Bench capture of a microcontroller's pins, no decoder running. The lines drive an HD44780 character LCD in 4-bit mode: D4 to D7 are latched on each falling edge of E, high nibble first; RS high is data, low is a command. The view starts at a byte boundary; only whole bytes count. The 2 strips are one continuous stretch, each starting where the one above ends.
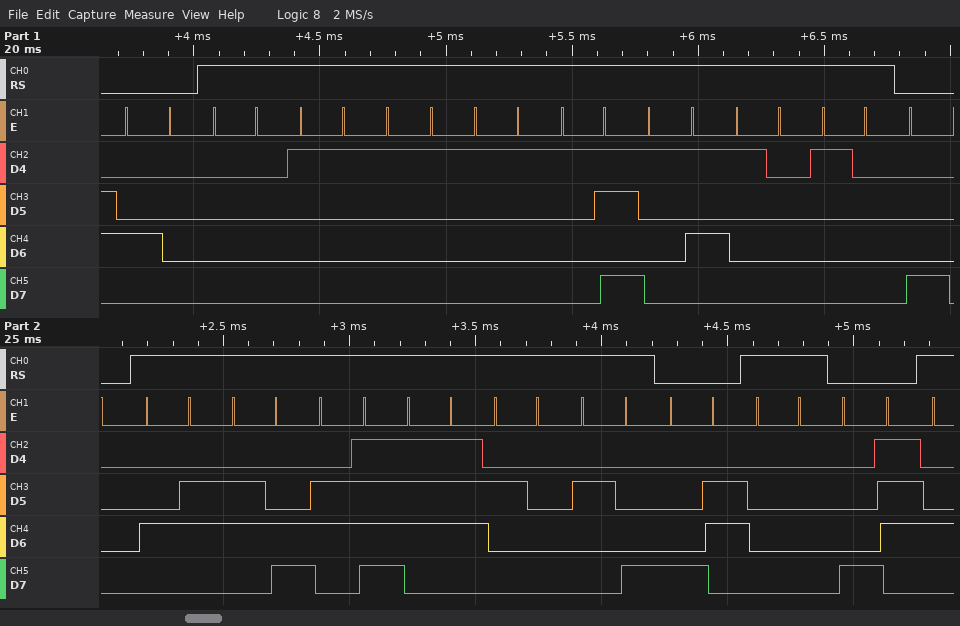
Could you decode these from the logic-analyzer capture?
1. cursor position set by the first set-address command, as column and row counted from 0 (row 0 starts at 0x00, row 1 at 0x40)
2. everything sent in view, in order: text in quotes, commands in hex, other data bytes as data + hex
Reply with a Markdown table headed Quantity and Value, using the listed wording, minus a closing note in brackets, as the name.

| Quantity | Value |
|---|---|
| cursor position set by the first set-address command, as column and row counted from 0 | column 0, row 0 |
| everything sent in view, in order: text in quotes, commands in hex, other data bytes as data + hex | 0x40 data 00 11 11 11 1B 15 10 10 0x80 "Flow (" 0x86 data 00 0x87 |
